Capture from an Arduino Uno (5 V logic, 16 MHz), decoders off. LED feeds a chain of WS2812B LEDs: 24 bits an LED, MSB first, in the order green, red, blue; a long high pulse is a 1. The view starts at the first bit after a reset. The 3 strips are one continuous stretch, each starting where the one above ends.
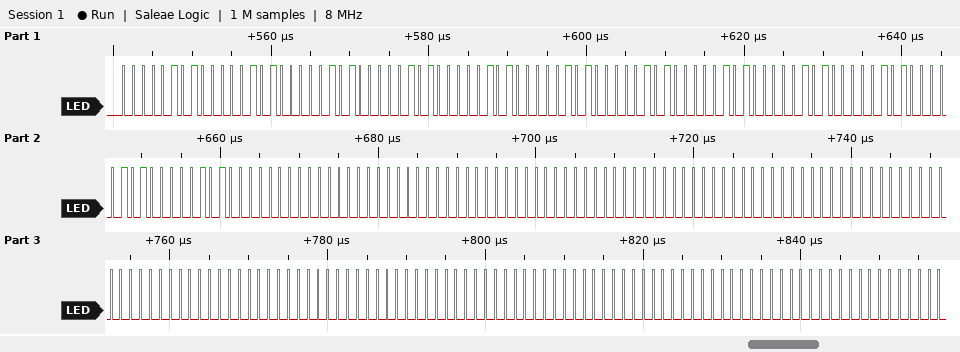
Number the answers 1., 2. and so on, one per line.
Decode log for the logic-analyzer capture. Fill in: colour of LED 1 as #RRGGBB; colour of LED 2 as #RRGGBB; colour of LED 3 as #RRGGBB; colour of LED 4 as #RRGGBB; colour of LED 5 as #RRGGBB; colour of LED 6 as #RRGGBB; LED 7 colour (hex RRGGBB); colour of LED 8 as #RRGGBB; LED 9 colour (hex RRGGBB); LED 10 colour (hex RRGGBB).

1. #050505
2. #050505
3. #050505
4. #050505
5. #000000
6. #000000
7. #000000
8. #000000
9. #000000
10. #000000
